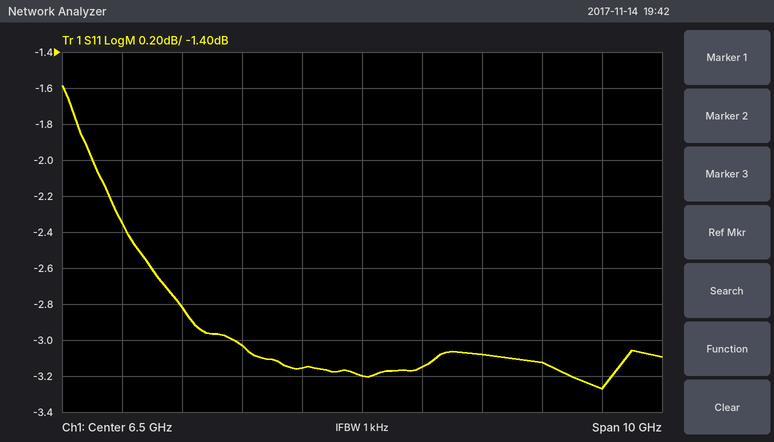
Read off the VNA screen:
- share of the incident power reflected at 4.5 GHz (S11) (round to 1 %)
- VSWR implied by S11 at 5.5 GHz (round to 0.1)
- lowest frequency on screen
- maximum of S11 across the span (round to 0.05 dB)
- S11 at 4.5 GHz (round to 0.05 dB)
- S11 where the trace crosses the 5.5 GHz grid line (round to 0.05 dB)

50 %
5.6
1.5 GHz
-1.60 dB
-3.05 dB
-3.15 dB
